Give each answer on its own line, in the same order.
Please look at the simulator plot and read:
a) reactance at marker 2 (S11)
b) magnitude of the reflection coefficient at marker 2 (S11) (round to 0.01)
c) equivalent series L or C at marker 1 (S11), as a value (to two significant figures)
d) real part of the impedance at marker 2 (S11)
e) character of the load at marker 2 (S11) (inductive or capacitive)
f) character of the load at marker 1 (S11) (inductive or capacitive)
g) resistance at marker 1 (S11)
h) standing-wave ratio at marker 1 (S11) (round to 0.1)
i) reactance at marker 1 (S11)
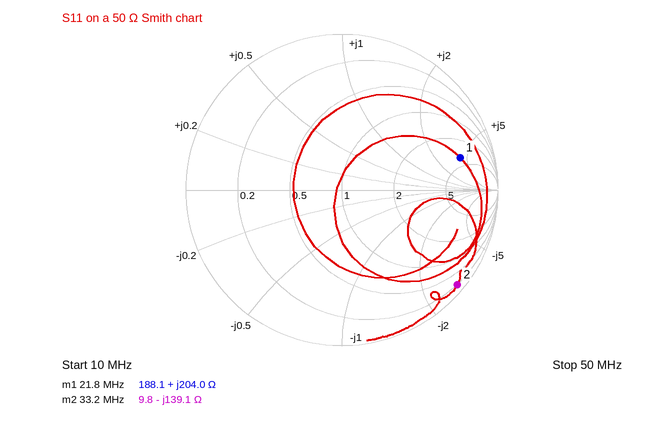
-139.1 Ω
0.96
1.5 µH
9.8 Ω
capacitive
inductive
188.1 Ω
8.3
+204.0 Ω
